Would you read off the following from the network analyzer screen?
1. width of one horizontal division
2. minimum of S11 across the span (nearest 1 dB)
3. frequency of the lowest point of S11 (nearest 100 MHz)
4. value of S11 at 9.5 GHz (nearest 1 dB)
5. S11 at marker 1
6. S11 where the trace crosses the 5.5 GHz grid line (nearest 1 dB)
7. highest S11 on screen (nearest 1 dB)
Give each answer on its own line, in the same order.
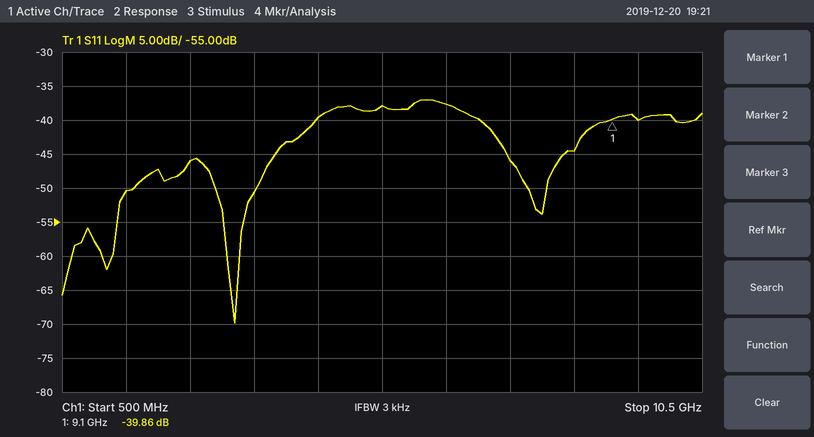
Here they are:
1 GHz
-70 dB
3.2 GHz
-40 dB
-39.86 dB
-38 dB
-37 dB
